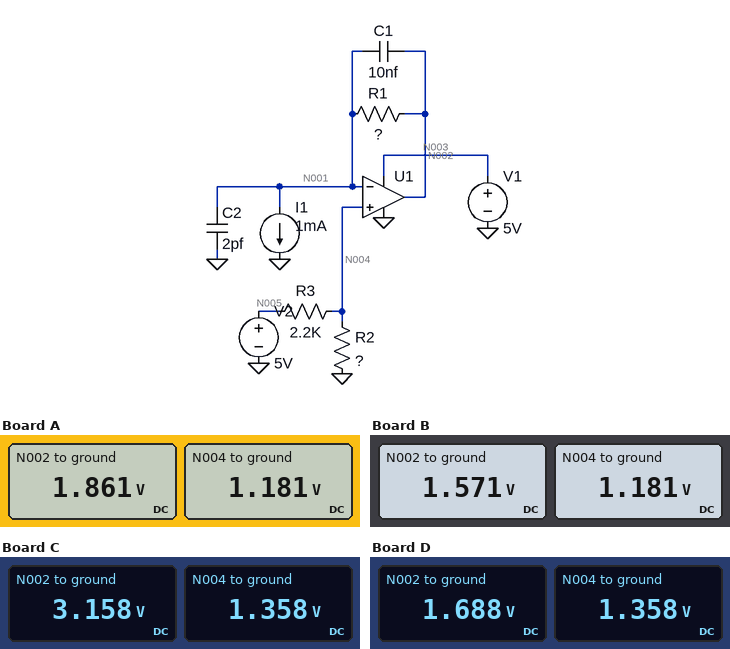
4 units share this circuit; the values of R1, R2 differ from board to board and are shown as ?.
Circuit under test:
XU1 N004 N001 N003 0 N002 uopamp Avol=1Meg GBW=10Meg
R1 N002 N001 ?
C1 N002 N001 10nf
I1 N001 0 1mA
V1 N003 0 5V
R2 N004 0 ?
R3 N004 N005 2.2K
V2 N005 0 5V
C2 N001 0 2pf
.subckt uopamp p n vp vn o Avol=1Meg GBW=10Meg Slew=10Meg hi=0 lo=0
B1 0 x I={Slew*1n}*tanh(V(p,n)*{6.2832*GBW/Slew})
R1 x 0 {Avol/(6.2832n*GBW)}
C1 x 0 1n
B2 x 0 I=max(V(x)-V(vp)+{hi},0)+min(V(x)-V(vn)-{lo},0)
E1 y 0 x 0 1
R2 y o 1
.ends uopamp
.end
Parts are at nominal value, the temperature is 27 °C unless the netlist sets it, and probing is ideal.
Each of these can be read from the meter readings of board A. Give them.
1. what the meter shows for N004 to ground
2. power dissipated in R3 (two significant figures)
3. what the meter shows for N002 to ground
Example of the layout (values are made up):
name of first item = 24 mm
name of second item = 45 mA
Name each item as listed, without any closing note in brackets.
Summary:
what the meter shows for N004 to ground = 1.181 V
power dissipated in R3 = 6.6 mW
what the meter shows for N002 to ground = 1.861 V
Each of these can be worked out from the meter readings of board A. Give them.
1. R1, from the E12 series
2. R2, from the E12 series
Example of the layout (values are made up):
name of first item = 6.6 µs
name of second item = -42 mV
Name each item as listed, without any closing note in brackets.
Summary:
R1, from the E12 series = 680 Ω
R2, from the E12 series = 680 Ω
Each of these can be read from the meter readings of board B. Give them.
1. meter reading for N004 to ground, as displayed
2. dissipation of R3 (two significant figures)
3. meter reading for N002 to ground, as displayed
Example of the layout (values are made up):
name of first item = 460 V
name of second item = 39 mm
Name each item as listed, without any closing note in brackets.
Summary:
meter reading for N004 to ground, as displayed = 1.181 V
dissipation of R3 = 6.6 mW
meter reading for N002 to ground, as displayed = 1.571 V
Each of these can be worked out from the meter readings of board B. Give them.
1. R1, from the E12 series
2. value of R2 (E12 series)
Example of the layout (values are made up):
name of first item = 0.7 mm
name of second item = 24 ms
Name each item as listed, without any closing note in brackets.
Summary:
R1, from the E12 series = 390 Ω
value of R2 = 680 Ω
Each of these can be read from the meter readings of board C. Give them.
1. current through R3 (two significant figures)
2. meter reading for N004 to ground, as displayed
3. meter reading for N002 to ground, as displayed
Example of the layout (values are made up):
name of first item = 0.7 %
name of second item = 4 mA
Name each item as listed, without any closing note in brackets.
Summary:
current through R3 = 1.7 mA
meter reading for N004 to ground, as displayed = 1.358 V
meter reading for N002 to ground, as displayed = 3.158 V
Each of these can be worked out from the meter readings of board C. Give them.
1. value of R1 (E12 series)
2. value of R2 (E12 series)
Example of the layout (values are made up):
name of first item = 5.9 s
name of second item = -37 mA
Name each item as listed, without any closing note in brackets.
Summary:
value of R1 = 1.8 kΩ
value of R2 = 820 Ω
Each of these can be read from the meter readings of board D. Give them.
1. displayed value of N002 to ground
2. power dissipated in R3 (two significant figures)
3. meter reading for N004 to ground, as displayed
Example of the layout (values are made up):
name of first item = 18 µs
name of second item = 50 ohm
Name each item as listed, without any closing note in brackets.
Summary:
displayed value of N002 to ground = 1.688 V
power dissipated in R3 = 6.0 mW
meter reading for N004 to ground, as displayed = 1.358 V
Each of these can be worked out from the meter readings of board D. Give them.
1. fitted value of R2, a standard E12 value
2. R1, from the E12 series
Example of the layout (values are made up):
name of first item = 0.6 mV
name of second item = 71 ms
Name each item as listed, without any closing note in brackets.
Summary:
fitted value of R2, a standard E12 value = 820 Ω
R1, from the E12 series = 330 Ω
